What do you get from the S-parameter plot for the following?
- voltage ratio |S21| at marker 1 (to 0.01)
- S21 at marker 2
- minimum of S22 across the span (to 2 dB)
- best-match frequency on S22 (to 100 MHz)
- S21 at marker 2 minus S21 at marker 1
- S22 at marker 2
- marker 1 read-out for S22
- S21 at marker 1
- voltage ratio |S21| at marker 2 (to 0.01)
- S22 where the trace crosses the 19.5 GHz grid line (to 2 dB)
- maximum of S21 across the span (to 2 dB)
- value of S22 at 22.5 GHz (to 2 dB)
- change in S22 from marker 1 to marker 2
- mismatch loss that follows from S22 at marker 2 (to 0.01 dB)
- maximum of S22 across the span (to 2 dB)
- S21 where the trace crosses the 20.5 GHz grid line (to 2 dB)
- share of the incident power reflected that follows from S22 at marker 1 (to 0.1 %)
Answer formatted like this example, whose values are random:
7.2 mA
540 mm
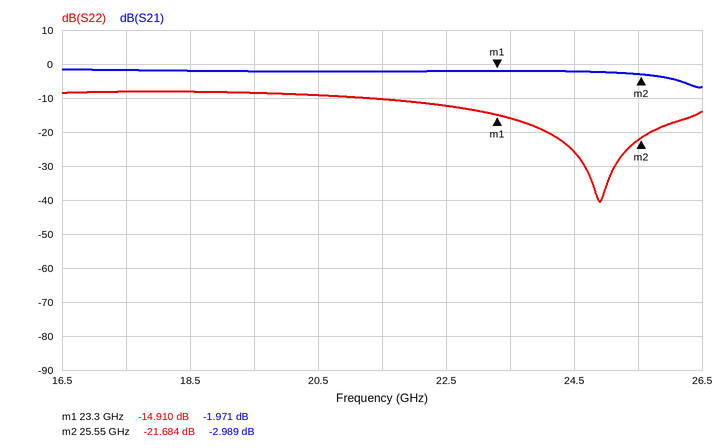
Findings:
0.80
-2.989 dB
-40 dB
24.9 GHz
-1.018 dB
-21.684 dB
-14.910 dB
-1.971 dB
0.71
-8 dB
-2 dB
-12 dB
-6.774 dB
0.03 dB
-8 dB
-2 dB
3.2 %
